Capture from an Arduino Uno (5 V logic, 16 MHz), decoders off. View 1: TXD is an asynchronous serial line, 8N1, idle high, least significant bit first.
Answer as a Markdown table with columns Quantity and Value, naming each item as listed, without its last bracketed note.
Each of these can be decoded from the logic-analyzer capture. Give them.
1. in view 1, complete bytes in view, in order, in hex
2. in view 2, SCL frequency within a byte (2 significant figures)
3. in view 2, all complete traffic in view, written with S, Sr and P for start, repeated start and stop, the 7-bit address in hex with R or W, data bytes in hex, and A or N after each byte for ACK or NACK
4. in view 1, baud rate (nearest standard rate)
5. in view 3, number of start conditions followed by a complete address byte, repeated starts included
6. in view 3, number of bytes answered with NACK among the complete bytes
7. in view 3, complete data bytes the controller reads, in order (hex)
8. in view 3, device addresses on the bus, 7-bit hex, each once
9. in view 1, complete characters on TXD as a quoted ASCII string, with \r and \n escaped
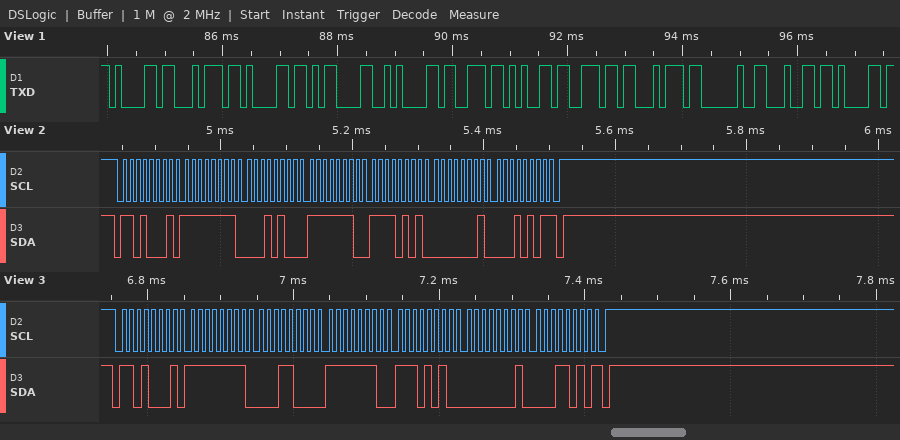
| Quantity | Value |
|---|---|
| in view 1, complete bytes in view, in order, in hex | 0x61 0x74 0x61 0x0D 0x0A 0x73 0x65 0x6E 0x74 0x20 0x64 0x61 |
| in view 2, SCL frequency within a byte | 100 kHz |
| in view 2, all complete traffic in view, written with S, Sr and P for start, repeated start and stop, the 7-bit address in hex with R or W, data bytes in hex, and A or N after each byte for ACK or NACK | S 68R A FF A 14 A FE A F5 A 01 A 15 N P |
| in view 1, baud rate | 9600 baud |
| in view 3, number of start conditions followed by a complete address byte, repeated starts included | 1 |
| in view 3, number of bytes answered with NACK among the complete bytes | 1 |
| in view 3, complete data bytes the controller reads, in order | FF 18 FE EA 01 1A |
| in view 3, device addresses on the bus, 7-bit hex, each once | 0x68 |
| in view 1, complete characters on TXD as a quoted ASCII string, with \r and \n escaped | "ata\r\nsent da" |
